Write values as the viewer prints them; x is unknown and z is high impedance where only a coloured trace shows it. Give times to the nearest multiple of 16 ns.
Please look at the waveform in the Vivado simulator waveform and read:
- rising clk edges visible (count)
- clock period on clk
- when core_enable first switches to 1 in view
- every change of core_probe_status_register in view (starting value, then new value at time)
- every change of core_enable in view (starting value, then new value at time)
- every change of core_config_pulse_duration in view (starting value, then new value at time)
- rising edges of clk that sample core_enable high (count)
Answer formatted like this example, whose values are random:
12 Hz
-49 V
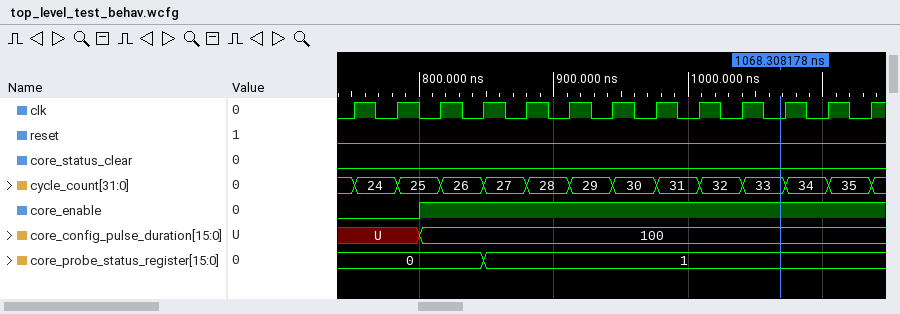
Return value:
13
32 ns
800 ns
0, 1 at 848 ns
0, 1 at 800 ns
U, 100 at 800 ns
11
